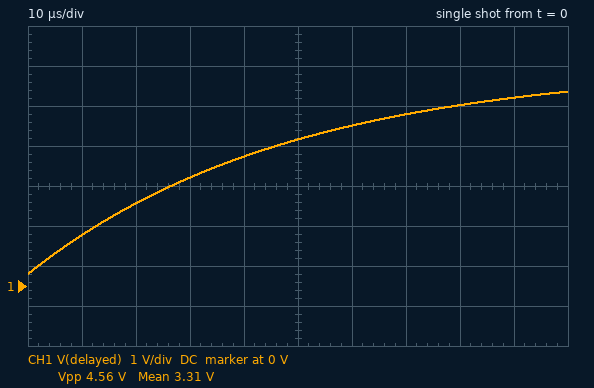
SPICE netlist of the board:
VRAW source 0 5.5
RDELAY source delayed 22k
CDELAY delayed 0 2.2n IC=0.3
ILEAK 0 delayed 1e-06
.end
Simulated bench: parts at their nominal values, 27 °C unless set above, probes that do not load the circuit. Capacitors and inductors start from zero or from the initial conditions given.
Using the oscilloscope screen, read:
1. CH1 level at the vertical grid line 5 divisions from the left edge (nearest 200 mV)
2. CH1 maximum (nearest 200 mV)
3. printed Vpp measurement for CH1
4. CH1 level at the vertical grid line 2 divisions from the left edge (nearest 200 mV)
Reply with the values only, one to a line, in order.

3.6 V
4.8 V
4.56 V
2.0 V
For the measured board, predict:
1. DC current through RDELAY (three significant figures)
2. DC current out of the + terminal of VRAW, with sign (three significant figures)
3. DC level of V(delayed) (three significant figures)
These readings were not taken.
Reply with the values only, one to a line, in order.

1.00 µA
-1.00 µA
5.52 V
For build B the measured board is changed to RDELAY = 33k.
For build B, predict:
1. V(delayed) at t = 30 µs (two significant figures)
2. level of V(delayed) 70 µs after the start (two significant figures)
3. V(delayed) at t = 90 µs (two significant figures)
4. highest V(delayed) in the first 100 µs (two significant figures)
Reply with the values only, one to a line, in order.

2.1 V
3.5 V
4.0 V
4.2 V
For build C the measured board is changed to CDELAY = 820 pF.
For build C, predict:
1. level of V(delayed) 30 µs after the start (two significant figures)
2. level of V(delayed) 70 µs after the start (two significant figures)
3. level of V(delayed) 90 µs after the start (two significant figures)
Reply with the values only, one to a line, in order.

4.5 V
5.4 V
5.5 V
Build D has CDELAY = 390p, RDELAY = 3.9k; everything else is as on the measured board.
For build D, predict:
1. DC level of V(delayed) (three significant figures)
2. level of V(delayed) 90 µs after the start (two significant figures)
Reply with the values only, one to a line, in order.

5.50 V
5.5 V
